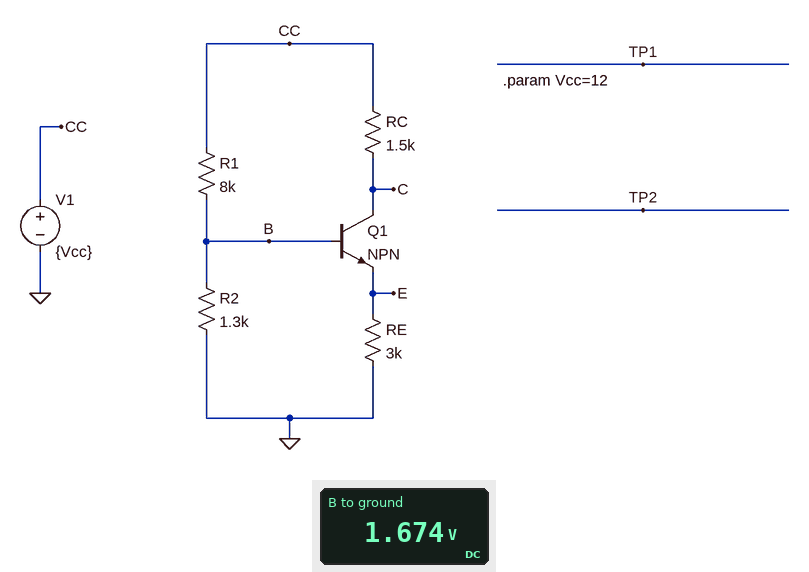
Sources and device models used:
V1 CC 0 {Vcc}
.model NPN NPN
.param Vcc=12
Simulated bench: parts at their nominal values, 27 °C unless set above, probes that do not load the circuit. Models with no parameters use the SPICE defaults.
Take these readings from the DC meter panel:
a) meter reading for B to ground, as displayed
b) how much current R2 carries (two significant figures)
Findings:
1.674 V
1.3 mA
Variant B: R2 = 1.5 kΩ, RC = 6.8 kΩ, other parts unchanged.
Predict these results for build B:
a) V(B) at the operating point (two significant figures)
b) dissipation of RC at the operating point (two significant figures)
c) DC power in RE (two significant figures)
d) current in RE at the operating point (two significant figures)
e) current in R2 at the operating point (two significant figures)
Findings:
1.9 V
960 µW
430 µW
380 µA
1.3 mA
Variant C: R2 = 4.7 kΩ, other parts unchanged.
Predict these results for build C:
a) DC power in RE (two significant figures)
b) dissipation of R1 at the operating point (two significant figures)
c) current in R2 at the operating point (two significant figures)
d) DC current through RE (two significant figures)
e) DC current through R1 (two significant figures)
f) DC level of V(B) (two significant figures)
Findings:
4.4 mW
7.2 mW
940 µA
1.2 mA
950 µA
4.4 V
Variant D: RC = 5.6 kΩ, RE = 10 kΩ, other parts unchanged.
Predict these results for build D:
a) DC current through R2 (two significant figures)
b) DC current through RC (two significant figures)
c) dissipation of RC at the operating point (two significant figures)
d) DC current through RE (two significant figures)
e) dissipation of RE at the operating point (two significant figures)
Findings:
1.3 mA
95 µA
51 µW
96 µA
93 µW
